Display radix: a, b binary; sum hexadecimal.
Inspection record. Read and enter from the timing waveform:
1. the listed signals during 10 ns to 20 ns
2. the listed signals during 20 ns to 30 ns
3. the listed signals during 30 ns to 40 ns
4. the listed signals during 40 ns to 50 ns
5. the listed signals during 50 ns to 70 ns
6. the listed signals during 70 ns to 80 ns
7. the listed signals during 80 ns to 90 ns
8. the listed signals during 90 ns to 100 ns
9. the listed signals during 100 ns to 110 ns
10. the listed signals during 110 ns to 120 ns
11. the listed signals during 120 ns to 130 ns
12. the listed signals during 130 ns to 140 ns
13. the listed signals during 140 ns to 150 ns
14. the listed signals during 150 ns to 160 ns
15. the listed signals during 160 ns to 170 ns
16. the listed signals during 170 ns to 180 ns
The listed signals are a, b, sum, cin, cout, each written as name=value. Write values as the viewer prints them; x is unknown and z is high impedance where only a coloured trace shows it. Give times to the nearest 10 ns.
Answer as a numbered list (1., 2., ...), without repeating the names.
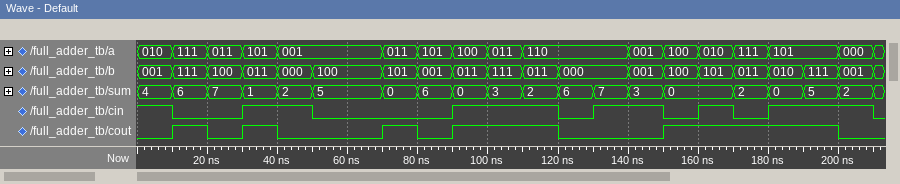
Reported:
1. a=111, b=111, sum=6, cin=0, cout=1
2. a=011, b=100, sum=7, cin=0, cout=0
3. a=101, b=011, sum=1, cin=1, cout=1
4. a=001, b=000, sum=2, cin=1, cout=0
5. a=001, b=100, sum=5, cin=0, cout=0
6. a=011, b=101, sum=0, cin=0, cout=1
7. a=101, b=001, sum=6, cin=0, cout=0
8. a=100, b=011, sum=0, cin=1, cout=1
9. a=011, b=111, sum=3, cin=1, cout=1
10. a=110, b=011, sum=2, cin=1, cout=1
11. a=110, b=000, sum=6, cin=0, cout=0
12. a=110, b=000, sum=7, cin=1, cout=0
13. a=001, b=001, sum=3, cin=1, cout=0
14. a=100, b=100, sum=0, cin=0, cout=1
15. a=010, b=101, sum=0, cin=1, cout=1
16. a=111, b=011, sum=2, cin=0, cout=1
